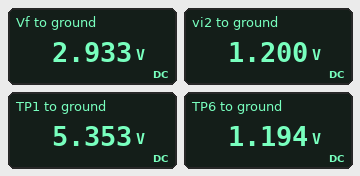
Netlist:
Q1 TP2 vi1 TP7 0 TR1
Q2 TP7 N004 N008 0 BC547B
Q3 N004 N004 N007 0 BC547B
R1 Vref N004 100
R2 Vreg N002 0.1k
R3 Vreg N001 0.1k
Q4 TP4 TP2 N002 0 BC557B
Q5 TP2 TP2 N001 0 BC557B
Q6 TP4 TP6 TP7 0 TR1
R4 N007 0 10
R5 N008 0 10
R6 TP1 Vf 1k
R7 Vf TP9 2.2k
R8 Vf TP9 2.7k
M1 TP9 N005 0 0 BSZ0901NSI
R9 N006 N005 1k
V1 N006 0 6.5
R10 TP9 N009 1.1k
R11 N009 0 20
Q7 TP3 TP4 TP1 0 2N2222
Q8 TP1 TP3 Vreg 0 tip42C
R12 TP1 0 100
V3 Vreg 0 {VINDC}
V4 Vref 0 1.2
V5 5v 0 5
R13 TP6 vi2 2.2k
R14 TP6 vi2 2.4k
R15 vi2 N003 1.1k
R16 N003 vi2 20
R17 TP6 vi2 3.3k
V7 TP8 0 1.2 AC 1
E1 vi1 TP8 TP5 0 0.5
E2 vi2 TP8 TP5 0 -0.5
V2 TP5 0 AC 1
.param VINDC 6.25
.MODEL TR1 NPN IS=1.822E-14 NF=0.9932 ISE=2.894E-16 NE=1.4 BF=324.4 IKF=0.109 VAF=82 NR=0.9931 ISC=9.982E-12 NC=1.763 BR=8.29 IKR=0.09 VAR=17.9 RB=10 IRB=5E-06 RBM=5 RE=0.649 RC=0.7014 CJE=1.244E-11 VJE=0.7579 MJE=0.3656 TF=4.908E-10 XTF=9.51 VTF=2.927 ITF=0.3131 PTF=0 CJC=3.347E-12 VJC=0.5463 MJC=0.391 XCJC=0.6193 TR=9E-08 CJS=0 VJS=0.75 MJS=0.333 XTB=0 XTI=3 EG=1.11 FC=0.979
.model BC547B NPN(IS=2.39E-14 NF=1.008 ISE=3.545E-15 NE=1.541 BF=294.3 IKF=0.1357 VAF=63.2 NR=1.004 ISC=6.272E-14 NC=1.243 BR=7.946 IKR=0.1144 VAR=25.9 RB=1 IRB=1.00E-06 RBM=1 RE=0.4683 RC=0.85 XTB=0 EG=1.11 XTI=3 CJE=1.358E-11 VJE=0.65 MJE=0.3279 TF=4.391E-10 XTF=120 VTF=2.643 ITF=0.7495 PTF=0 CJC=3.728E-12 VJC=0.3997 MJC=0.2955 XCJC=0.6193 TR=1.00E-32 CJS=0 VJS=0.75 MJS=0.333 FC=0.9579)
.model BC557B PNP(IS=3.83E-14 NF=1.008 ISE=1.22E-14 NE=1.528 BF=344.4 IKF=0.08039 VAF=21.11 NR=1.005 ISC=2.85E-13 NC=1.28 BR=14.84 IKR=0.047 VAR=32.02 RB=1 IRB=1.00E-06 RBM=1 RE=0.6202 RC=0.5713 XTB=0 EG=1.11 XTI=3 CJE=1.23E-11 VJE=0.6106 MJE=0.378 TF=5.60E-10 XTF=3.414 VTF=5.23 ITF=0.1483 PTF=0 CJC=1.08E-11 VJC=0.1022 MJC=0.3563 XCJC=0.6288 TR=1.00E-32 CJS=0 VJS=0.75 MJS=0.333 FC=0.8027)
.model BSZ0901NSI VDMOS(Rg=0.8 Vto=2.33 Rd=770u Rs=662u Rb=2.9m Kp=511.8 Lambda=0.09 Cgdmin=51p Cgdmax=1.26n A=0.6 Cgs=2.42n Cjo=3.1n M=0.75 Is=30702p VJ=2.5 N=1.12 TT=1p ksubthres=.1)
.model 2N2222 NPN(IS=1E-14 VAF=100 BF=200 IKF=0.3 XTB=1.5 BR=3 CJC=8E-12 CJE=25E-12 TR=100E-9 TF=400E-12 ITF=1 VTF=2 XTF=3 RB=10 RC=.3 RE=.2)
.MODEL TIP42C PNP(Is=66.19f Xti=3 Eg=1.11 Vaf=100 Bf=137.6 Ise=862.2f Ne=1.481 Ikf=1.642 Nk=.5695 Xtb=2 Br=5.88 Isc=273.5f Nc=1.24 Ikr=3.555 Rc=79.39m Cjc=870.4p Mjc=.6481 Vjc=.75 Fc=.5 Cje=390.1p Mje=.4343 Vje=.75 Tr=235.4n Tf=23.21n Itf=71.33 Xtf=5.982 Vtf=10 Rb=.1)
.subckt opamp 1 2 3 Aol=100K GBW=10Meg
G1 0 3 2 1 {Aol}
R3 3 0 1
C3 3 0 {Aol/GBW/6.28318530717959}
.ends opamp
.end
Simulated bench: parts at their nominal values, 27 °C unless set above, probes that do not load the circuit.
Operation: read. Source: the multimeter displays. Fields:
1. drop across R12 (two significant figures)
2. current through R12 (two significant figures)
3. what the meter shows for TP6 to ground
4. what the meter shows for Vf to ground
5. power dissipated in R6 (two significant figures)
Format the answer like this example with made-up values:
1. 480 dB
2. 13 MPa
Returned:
1. 5.4 V
2. 54 mA
3. 1.194 V
4. 2.933 V
5. 5.9 mW
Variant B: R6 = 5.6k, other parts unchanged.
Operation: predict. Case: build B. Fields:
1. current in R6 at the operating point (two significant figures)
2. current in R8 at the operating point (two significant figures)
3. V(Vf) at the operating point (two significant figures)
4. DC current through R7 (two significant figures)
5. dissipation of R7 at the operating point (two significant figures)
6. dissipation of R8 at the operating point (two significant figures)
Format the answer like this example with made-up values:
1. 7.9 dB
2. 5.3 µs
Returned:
1. 790 µA
2. 350 µA
3. 950 mV
4. 430 µA
5. 410 µW
6. 340 µW
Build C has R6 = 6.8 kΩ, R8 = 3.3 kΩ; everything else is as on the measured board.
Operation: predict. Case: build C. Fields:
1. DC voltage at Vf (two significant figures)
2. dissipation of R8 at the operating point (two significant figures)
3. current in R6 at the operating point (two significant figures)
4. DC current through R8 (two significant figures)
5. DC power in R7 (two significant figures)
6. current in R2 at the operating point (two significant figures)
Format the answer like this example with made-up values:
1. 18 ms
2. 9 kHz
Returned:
1. 870 mV
2. 230 µW
3. 660 µA
4. 260 µA
5. 340 µW
6. 2.3 mA
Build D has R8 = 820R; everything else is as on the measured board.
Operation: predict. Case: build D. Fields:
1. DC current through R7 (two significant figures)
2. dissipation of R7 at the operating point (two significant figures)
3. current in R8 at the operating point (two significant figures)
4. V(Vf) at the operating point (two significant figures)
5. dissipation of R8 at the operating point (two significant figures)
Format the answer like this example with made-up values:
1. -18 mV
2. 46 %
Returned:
1. 910 µA
2. 1.8 mW
3. 2.4 mA
4. 2.0 V
5. 4.9 mW
